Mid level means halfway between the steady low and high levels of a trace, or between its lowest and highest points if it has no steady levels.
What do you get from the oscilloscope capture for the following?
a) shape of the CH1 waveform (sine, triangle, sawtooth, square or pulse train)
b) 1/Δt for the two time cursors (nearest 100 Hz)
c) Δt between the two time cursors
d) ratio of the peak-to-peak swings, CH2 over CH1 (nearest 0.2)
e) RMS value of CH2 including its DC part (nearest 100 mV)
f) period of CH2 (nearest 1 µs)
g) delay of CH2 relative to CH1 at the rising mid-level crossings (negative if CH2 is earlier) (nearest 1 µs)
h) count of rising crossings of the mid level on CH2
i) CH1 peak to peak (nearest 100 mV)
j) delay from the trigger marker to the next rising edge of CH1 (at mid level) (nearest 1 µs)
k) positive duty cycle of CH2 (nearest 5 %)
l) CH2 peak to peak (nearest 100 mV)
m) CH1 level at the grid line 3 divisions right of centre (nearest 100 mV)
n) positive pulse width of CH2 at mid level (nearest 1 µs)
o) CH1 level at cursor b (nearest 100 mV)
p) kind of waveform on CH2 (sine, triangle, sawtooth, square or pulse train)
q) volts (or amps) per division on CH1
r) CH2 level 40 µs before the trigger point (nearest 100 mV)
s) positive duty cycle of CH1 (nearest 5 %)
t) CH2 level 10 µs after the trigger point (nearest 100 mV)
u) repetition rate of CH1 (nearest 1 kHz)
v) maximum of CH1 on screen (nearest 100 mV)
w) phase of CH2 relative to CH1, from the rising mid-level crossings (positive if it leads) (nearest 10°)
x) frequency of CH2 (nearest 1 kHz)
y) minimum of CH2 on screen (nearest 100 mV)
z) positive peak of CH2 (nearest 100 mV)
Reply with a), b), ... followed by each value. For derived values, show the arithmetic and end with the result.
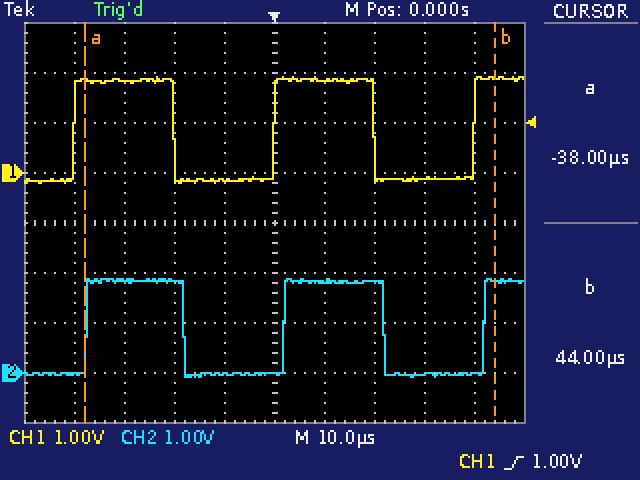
a) square
b) 1 / 82 µs ≈ 12.2 kHz
c) 44 µs − (-38 µs) = 82 µs
d) 2.0 V / 2.1 V ≈ 1.0
e) √(0.5 × (1.9 V)² + 0.5 × (-100 mV)²) ≈ 1.3 V
f) 40 µs
g) +2 µs
h) 3
i) 1.9 V − (-200 mV) = 2.1 V
j) 40 µs
k) 20 µs / 40 µs ≈ 50 %
l) 1.9 V − (-100 mV) = 2.0 V
m) -100 mV
n) 20 µs
o) 1.9 V
p) square
q) 1 V
r) 0.0 V
s) 20 µs / 40 µs ≈ 50 %
t) 1.8 V
u) 1 / 40 µs ≈ 25 kHz
v) 1.9 V
w) −360° × (+2 µs) / 40 µs ≈ -18.0°, so -20° to the nearest 10°
x) 1 / 40 µs ≈ 25 kHz
y) -100 mV
z) 1.9 V
